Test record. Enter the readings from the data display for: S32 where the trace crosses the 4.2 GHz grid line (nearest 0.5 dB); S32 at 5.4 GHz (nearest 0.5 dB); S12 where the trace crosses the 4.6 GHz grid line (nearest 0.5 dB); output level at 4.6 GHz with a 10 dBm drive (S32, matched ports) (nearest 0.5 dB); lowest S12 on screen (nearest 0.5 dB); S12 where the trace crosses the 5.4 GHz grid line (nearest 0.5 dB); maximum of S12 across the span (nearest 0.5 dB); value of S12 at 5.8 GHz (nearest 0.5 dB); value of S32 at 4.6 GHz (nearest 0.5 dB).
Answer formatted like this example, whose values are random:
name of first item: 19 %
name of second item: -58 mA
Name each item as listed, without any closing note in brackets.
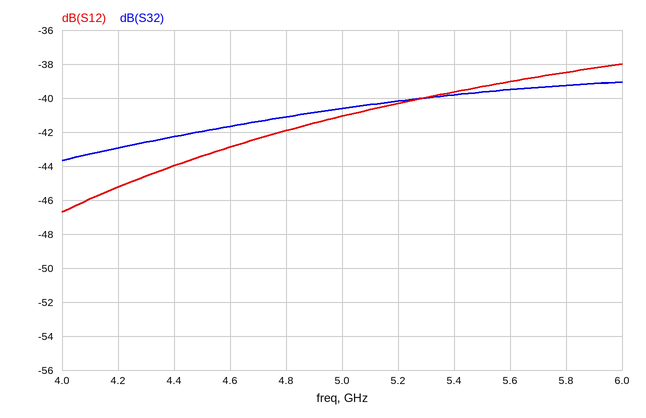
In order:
S32 where the trace crosses the 4.2 GHz grid line: -43.0 dB
S32 at 5.4 GHz: -40.0 dB
S12 where the trace crosses the 4.6 GHz grid line: -43.0 dB
output level at 4.6 GHz with a 10 dBm drive (S32, matched ports): -31.5 dBm
lowest S12 on screen: -46.5 dB
S12 where the trace crosses the 5.4 GHz grid line: -39.5 dB
maximum of S12 across the span: -38.0 dB
value of S12 at 5.8 GHz: -38.5 dB
value of S32 at 4.6 GHz: -41.5 dB
